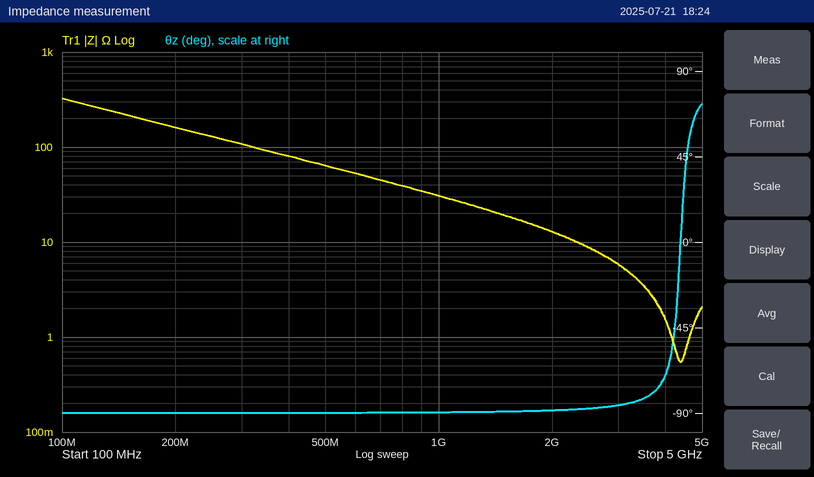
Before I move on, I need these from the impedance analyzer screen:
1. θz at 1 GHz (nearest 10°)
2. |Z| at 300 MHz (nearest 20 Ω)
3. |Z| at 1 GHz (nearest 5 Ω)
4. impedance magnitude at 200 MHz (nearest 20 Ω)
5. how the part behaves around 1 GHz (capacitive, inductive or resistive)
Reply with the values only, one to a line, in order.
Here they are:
-90°
100 Ω
30 Ω
160 Ω
capacitive
